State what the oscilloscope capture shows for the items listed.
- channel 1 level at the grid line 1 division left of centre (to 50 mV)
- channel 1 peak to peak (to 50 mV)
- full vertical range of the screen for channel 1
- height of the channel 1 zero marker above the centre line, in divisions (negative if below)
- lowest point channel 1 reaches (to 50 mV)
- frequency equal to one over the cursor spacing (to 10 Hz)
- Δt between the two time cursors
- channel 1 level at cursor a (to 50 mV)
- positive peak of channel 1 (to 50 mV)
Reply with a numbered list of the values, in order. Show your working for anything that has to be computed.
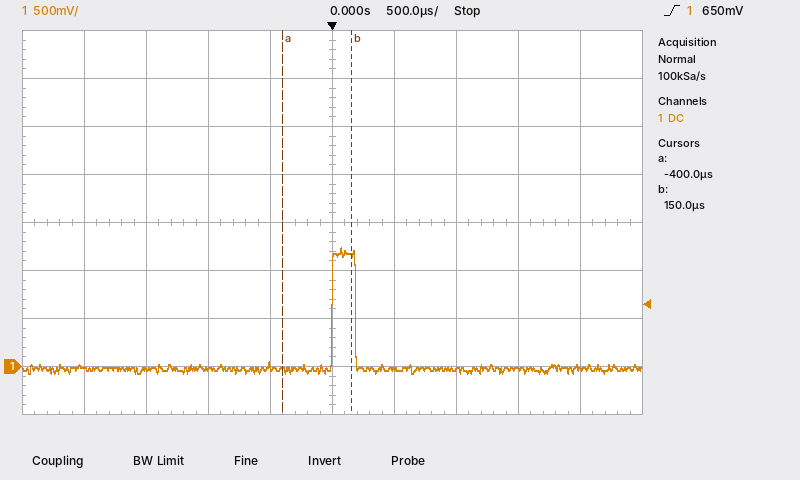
1. 0 mV
2. 1.25 V − (-50 mV) = 1.30 V
3. 4 V
4. -3.0 div
5. -50 mV
6. 1 / 550 µs ≈ 1.82 kHz
7. 150 µs − (-400 µs) = 550 µs
8. -50 mV
9. 1.25 V
